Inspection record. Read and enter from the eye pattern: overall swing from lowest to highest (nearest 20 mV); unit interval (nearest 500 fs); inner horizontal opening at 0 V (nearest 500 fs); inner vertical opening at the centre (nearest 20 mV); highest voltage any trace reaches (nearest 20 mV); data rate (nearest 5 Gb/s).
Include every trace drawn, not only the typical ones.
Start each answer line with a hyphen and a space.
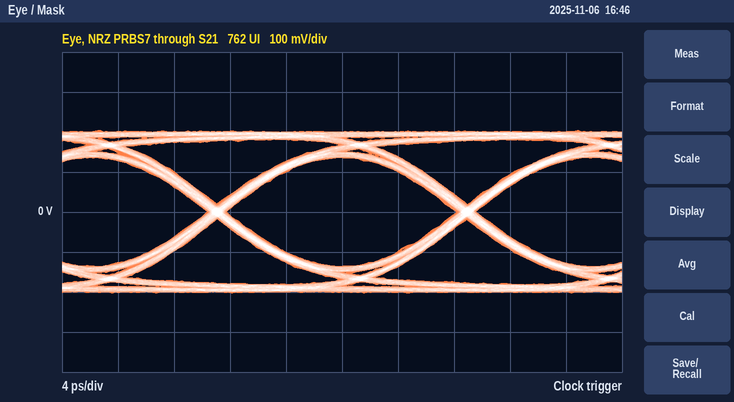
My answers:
- 400 mV
- 18.0 ps
- 16.5 ps
- 280 mV
- 200 mV
- 55 Gb/s
